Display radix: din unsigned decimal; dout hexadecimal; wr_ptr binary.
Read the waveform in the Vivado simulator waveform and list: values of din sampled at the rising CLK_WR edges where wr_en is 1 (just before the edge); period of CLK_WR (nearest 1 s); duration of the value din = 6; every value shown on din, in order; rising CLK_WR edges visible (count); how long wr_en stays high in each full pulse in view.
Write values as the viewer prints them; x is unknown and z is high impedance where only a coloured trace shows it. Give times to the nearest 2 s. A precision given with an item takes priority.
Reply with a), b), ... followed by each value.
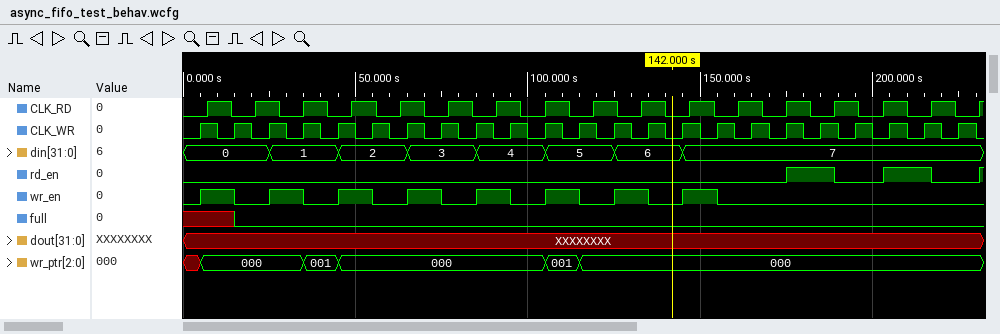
a) 0, 1, 2, 3, 4, 5, 6, 7
b) 10 s
c) 20 s
d) 0, 1, 2, 3, 4, 5, 6, 7
e) 23
f) 10 s, 10 s, 10 s, 10 s, 10 s, 10 s, 10 s, 10 s
